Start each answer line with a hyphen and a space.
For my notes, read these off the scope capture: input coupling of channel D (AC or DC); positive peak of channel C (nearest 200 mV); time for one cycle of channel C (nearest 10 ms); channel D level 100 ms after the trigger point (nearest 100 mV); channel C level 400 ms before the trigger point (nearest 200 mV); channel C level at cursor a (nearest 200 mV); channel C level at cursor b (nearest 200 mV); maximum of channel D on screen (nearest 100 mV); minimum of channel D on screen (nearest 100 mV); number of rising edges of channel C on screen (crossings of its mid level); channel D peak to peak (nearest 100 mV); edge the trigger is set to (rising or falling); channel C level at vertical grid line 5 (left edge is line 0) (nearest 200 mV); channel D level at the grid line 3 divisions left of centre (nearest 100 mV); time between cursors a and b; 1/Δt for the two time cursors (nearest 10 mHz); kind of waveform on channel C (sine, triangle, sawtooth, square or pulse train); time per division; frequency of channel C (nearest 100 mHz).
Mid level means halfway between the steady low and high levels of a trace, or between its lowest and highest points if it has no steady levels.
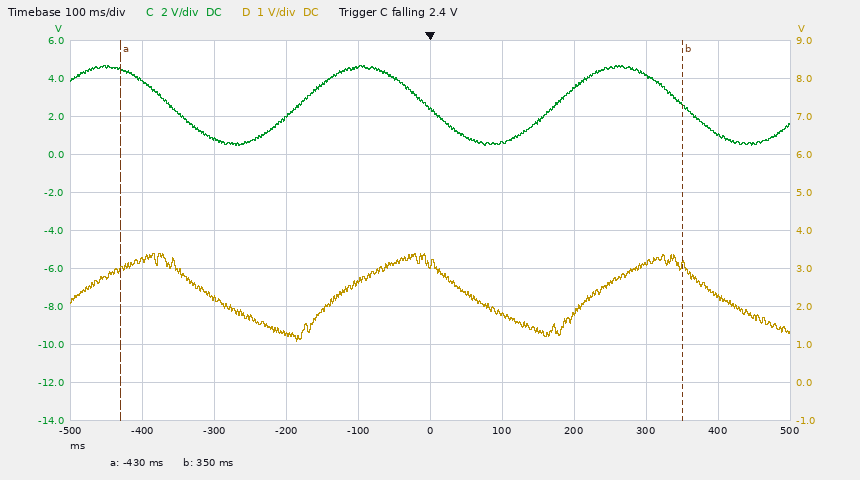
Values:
- DC
- 4.6 V
- 360 ms
- 1.8 V
- 3.8 V
- 4.4 V
- 2.6 V
- 3.4 V
- 1.1 V
- 2
- 2.3 V
- falling
- 2.4 V
- 2.2 V
- 780 ms
- 1.28 Hz
- sine
- 100 ms
- 2.8 Hz
